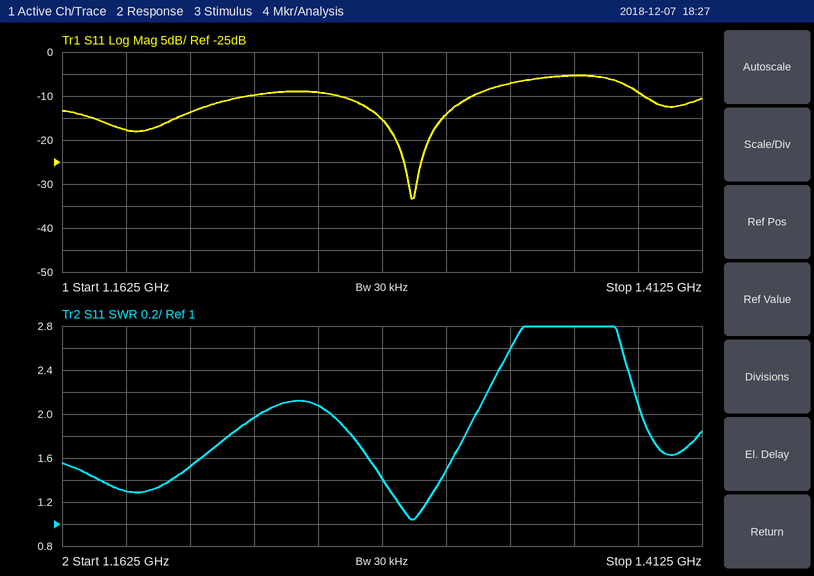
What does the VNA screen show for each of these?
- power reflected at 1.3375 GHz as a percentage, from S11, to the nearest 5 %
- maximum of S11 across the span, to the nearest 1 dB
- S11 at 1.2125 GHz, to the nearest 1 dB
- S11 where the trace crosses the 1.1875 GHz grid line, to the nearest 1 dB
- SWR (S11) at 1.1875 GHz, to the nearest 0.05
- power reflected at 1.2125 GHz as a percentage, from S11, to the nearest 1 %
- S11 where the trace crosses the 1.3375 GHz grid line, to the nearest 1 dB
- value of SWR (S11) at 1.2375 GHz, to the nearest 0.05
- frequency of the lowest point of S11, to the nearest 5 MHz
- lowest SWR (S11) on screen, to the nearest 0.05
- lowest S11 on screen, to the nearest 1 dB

20 %
-5 dB
-14 dB
-18 dB
1.30
4 %
-7 dB
1.95
1.300 GHz
1.05
-33 dB
